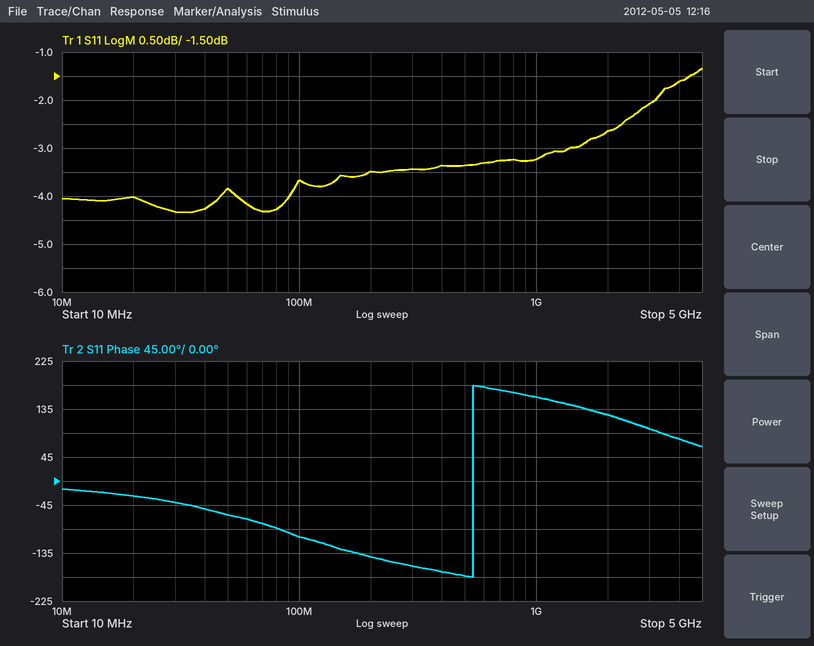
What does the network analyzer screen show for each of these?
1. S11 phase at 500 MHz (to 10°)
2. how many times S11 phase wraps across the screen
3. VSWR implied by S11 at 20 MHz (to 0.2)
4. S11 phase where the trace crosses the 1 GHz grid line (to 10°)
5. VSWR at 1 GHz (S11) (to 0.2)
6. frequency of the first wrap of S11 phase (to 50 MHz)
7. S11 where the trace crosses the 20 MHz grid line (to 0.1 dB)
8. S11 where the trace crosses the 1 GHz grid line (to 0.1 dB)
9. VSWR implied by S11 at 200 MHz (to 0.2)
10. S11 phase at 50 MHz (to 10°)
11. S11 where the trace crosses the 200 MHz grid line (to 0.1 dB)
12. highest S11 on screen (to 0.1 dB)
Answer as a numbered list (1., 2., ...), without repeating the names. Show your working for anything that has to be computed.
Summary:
1. -180°
2. 1
3. |Γ| = 10^(-4/20) = 0.6310; VSWR = (1 + 0.6310)/(1 − 0.6310) ≈ 4.4
4. 160°
5. |Γ| = 10^(-3.2/20) = 0.6918; VSWR = (1 + 0.6918)/(1 − 0.6918) ≈ 5.49, so 5.4 to the nearest 0.2
6. 550 MHz
7. -4.0 dB
8. -3.2 dB
9. |Γ| = 10^(-3.5/20) = 0.6683; VSWR = (1 + 0.6683)/(1 − 0.6683) ≈ 5.0
10. -60°
11. -3.5 dB
12. -1.3 dB
